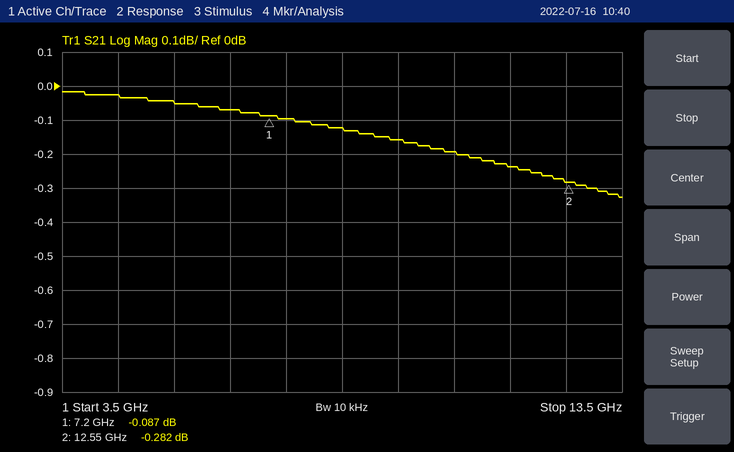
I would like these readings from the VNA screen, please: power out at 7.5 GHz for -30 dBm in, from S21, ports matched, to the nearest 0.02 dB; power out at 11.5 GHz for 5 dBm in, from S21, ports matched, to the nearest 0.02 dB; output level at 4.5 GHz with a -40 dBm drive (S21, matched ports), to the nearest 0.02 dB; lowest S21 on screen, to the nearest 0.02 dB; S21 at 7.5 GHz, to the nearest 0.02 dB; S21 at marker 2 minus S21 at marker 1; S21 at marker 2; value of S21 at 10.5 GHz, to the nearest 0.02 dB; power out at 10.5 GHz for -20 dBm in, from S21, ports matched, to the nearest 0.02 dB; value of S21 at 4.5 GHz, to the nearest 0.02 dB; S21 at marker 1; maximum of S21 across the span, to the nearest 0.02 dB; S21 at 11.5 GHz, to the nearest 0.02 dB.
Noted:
-30.10 dBm
4.76 dBm
-40.02 dBm
-0.32 dB
-0.10 dB
-0.195 dB
-0.282 dB
-0.20 dB
-20.20 dBm
-0.02 dB
-0.087 dB
-0.02 dB
-0.24 dB
